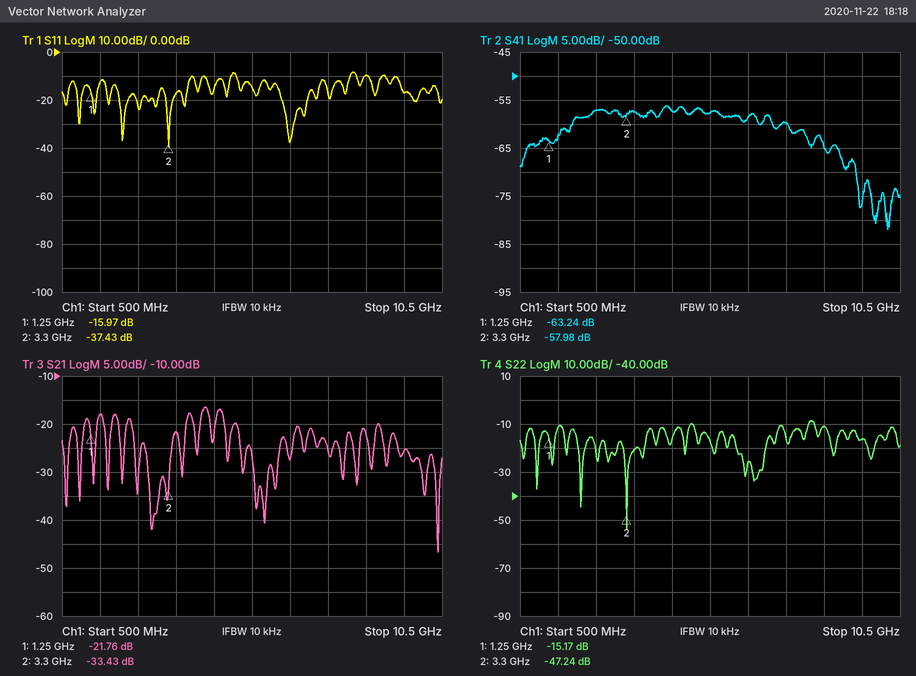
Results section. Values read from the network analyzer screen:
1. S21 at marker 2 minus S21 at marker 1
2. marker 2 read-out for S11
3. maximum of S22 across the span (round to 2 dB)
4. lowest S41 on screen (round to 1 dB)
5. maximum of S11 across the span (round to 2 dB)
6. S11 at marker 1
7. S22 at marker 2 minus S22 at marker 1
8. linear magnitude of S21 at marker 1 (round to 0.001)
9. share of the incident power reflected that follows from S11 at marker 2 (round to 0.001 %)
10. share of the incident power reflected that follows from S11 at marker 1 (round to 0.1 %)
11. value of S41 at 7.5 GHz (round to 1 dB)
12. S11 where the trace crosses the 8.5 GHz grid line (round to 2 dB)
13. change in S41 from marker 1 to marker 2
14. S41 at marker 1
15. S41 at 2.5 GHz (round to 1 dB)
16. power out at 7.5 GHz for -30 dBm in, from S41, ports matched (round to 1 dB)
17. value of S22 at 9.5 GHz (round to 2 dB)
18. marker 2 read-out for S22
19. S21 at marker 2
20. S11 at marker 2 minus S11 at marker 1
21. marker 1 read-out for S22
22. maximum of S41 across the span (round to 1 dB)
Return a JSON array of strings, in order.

["-11.67 dB", "-37.43 dB", "-8 dB", "-82 dB", "-8 dB", "-15.97 dB", "-32.07 dB", "0.082", "0.018 %", "2.5 %", "-60 dB", "-10 dB", "5.26 dB", "-63.24 dB", "-57 dB", "-90 dBm", "-16 dB", "-47.24 dB", "-33.43 dB", "-21.46 dB", "-15.17 dB", "-56 dB"]
